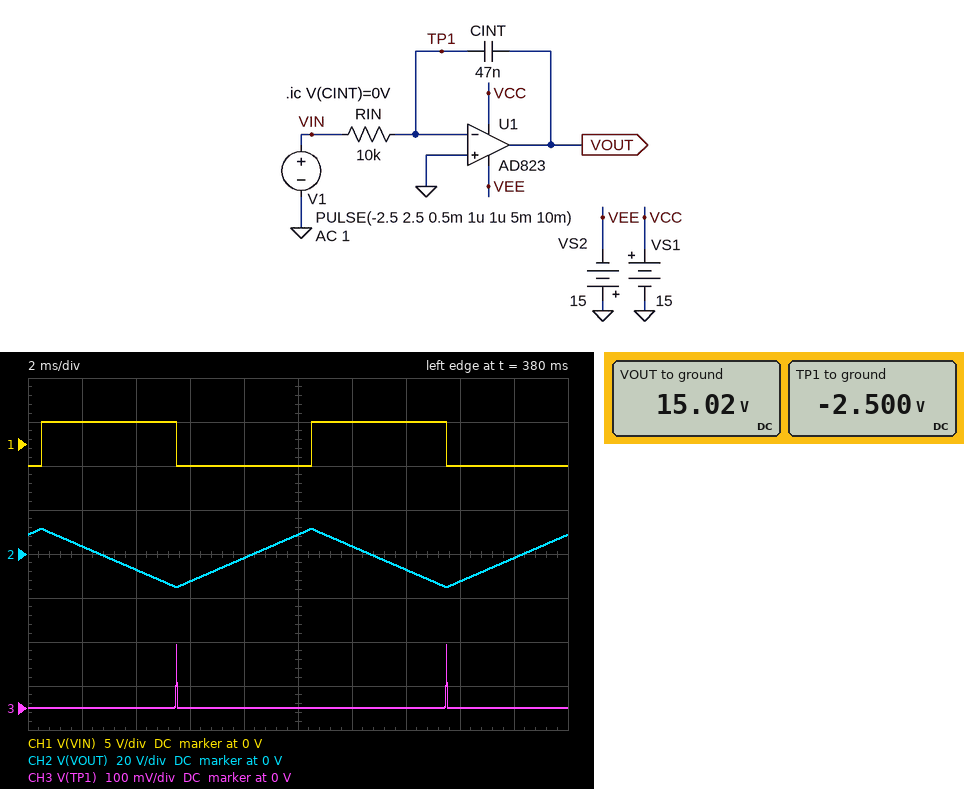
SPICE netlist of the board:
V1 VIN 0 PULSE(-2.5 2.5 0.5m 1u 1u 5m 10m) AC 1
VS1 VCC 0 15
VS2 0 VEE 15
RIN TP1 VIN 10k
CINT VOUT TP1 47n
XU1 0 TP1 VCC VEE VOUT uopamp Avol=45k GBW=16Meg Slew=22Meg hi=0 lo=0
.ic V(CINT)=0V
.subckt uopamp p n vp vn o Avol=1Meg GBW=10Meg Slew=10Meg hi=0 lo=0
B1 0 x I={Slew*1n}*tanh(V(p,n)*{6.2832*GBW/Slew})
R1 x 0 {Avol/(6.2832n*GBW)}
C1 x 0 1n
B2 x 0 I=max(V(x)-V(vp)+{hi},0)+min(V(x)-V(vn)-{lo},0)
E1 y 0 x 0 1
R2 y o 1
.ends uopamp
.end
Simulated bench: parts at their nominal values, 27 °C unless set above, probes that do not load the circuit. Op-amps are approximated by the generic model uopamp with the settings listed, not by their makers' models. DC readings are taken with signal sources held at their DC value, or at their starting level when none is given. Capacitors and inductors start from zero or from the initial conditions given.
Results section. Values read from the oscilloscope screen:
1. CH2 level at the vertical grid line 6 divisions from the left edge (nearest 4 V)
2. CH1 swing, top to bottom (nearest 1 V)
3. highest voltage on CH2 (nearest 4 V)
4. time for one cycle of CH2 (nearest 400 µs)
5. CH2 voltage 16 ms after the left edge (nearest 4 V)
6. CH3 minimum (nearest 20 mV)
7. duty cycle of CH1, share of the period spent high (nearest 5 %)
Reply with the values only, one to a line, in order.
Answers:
4 V
5 V
12 V
10.0 ms
-12 V
0 V
50 %
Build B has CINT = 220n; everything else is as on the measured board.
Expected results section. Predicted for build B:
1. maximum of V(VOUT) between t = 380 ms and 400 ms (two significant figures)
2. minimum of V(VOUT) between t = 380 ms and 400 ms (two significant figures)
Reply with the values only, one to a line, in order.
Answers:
490 mV
-5.2 V
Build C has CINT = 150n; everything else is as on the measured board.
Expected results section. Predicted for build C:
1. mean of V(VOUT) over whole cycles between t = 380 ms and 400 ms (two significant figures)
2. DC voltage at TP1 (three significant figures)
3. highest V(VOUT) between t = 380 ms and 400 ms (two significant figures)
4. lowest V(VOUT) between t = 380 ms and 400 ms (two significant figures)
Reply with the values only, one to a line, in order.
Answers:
-3.4 V
-2.50 V
720 mV
-7.6 V
